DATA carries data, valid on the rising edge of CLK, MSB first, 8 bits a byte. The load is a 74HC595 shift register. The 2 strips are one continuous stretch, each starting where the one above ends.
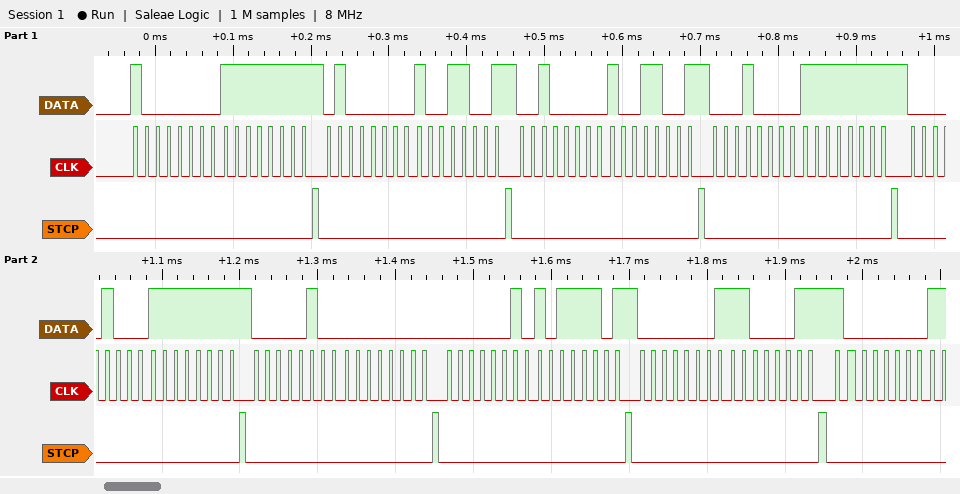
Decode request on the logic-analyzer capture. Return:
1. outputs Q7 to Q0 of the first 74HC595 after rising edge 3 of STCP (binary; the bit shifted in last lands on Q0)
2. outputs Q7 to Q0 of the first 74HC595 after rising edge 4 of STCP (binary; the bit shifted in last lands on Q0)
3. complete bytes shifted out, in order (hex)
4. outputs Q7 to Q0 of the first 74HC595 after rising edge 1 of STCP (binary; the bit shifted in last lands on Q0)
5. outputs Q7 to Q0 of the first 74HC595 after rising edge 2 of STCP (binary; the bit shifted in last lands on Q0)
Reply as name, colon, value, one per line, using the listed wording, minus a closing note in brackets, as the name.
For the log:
outputs Q7 to Q0 of the first 74HC595 after rising edge 3 of STCP: 10011001
outputs Q7 to Q0 of the first 74HC595 after rising edge 4 of STCP: 11111111
complete bytes shifted out, in order: 80 FF 40 99 20 99 10 FF 08 FF 04 00 02 BD 01 C3 80
outputs Q7 to Q0 of the first 74HC595 after rising edge 1 of STCP: 11111111
outputs Q7 to Q0 of the first 74HC595 after rising edge 2 of STCP: 10011001
